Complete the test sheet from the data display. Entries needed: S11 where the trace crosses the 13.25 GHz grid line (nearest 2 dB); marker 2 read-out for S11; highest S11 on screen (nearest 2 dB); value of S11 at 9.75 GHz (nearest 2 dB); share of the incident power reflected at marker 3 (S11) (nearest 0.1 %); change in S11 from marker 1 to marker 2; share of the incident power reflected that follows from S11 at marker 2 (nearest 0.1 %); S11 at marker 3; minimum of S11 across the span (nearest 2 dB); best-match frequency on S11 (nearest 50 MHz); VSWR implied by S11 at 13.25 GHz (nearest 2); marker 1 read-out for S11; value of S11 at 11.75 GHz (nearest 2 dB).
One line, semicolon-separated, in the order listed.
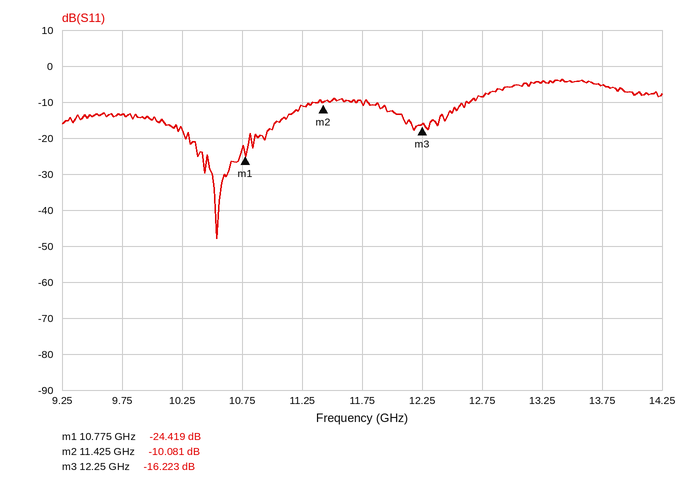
-4 dB; -10.081 dB; -4 dB; -14 dB; 2.4 %; 14.338 dB; 9.8 %; -16.223 dB; -48 dB; 10.55 GHz; 4; -24.419 dB; -10 dB
